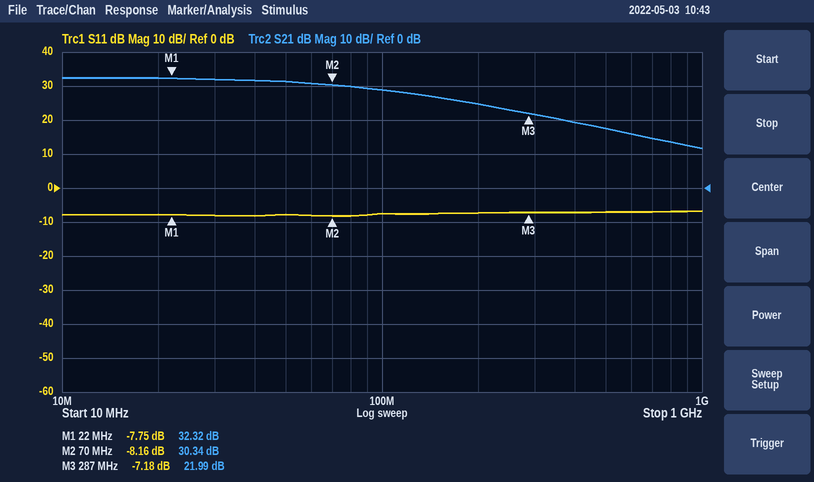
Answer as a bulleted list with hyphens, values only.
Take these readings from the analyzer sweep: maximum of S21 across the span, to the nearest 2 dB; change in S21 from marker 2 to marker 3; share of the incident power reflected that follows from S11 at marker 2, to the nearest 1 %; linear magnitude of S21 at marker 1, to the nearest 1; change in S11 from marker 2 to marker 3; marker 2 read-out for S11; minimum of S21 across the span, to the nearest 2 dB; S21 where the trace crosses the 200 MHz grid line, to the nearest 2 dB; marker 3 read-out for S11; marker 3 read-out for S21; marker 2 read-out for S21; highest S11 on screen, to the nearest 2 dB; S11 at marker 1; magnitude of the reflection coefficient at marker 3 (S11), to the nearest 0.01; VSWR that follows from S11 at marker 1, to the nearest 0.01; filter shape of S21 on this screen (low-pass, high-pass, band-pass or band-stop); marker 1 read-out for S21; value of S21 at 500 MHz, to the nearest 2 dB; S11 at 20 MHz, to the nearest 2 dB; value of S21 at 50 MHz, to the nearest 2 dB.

- 32 dB
- -8.35 dB
- 15 %
- 41
- 0.98 dB
- -8.16 dB
- 12 dB
- 24 dB
- -7.18 dB
- 21.99 dB
- 30.34 dB
- -6 dB
- -7.75 dB
- 0.44
- 2.39
- low-pass
- 32.32 dB
- 18 dB
- -8 dB
- 32 dB
